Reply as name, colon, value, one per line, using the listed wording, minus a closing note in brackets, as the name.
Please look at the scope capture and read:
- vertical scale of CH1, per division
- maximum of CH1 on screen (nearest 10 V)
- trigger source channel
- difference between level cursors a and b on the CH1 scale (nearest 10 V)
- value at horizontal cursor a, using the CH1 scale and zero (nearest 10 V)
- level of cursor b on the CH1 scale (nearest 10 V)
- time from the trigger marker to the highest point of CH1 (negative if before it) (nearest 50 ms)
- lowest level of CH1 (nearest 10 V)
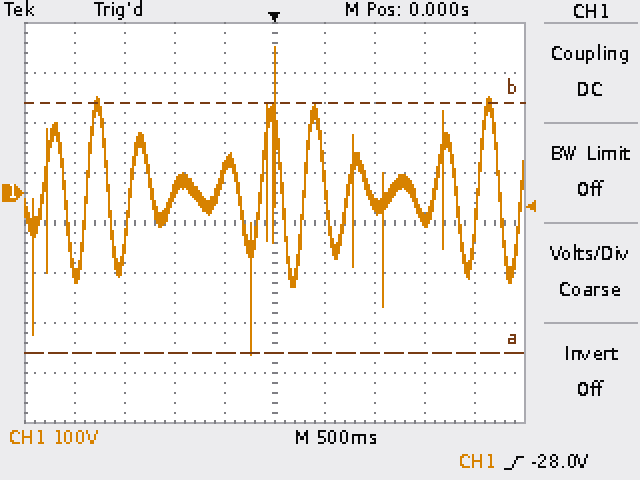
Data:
vertical scale of CH1, per division: 100 V
maximum of CH1 on screen: 290 V
trigger source channel: CH1
difference between level cursors a and b on the CH1 scale: 500 V
value at horizontal cursor a, using the CH1 scale and zero: -320 V
level of cursor b on the CH1 scale: 180 V
time from the trigger marker to the highest point of CH1 (negative if before it): 0 ms
lowest level of CH1: -320 V
